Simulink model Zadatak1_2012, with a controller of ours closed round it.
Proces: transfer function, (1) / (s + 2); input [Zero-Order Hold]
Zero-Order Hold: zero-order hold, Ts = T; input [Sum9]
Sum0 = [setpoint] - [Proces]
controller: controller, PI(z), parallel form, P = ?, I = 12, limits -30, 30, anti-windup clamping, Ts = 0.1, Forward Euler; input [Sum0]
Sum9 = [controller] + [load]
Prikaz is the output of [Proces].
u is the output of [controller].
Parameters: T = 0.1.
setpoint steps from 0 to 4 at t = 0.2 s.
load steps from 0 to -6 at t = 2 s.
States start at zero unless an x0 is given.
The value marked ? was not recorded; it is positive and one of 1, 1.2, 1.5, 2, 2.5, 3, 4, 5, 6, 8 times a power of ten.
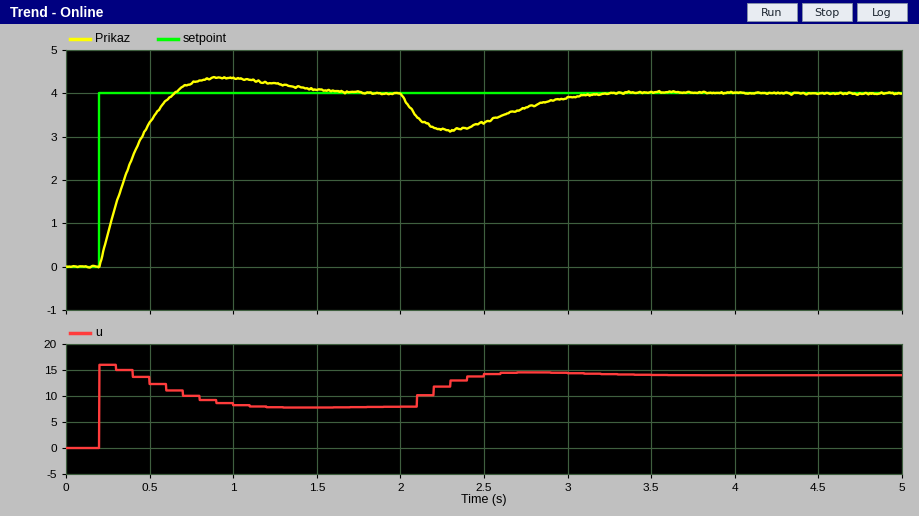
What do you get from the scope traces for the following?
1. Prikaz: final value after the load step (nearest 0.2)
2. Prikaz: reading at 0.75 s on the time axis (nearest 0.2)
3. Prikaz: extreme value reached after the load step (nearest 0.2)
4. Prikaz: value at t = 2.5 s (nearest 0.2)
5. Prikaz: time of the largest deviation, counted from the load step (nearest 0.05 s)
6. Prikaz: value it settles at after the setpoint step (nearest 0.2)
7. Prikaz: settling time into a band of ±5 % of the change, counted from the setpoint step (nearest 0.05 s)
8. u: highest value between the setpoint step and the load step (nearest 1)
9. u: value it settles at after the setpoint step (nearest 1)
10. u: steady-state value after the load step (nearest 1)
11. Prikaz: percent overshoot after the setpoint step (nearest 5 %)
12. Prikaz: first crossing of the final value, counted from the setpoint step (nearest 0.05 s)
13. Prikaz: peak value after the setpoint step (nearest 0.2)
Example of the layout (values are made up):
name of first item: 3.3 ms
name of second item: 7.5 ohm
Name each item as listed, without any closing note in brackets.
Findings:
Prikaz: final value after the load step: 4.0
Prikaz: reading at 0.75 s on the time axis: 4.2
Prikaz: extreme value reached after the load step: 3.2
Prikaz: value at t = 2.5 s: 3.4
Prikaz: time of the largest deviation, counted from the load step: 0.30 s
Prikaz: value it settles at after the setpoint step: 4.0
Prikaz: settling time into a band of ±5 % of the change, counted from the setpoint step: 1.10 s
u: highest value between the setpoint step and the load step: 16
u: value it settles at after the setpoint step: 8
u: steady-state value after the load step: 14
Prikaz: percent overshoot after the setpoint step: 10 %
Prikaz: first crossing of the final value, counted from the setpoint step: 0.45 s
Prikaz: peak value after the setpoint step: 4.4
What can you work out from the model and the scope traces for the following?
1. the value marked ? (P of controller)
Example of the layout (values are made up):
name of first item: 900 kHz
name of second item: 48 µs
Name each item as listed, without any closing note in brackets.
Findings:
the value marked ?: 4
